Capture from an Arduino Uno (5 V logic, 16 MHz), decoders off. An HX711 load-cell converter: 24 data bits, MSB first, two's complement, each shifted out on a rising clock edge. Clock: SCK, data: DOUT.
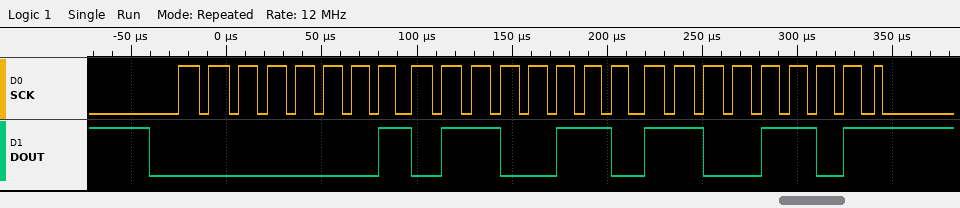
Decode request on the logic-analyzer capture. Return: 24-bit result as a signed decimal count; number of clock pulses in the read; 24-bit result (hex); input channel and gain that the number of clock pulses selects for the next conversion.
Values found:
91853
25
0x0166CD
channel A, gain 128
